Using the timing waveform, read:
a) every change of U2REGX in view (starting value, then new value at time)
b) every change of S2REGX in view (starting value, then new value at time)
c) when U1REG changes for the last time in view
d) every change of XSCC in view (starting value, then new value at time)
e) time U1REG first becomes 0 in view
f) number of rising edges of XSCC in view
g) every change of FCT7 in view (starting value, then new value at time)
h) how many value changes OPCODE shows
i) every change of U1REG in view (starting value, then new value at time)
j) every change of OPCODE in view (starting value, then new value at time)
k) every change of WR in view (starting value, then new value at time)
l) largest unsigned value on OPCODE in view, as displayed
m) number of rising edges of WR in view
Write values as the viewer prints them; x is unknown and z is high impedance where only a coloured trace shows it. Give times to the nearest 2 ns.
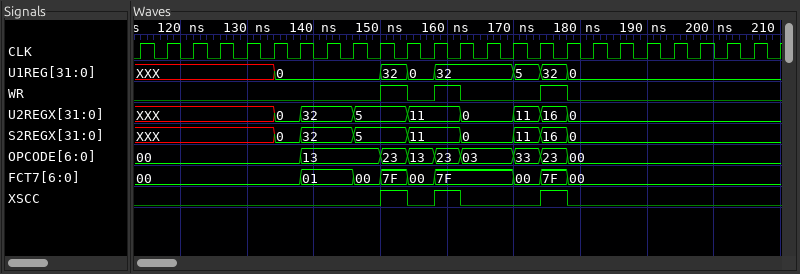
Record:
XXX, 0 at 134 ns, 32 at 138 ns, 5 at 146 ns, 11 at 154 ns, 0 at 162 ns, 11 at 170 ns, 16 at 174 ns, 0 at 178 ns
XXX, 0 at 134 ns, 32 at 138 ns, 5 at 146 ns, 11 at 154 ns, 0 at 162 ns, 11 at 170 ns, 16 at 174 ns, 0 at 178 ns
178 ns
0, 1 at 150 ns, 0 at 154 ns, 1 at 158 ns, 0 at 162 ns, 1 at 174 ns, 0 at 178 ns
134 ns
3
00, 01 at 138 ns, 00 at 146 ns, 7F at 150 ns, 00 at 154 ns, 7F at 158 ns, 00 at 170 ns, 7F at 174 ns, 00 at 178 ns
8
XXX, 0 at 134 ns, 32 at 150 ns, 0 at 154 ns, 32 at 158 ns, 5 at 170 ns, 32 at 174 ns, 0 at 178 ns
00, 13 at 138 ns, 23 at 150 ns, 13 at 154 ns, 23 at 158 ns, 03 at 162 ns, 33 at 170 ns, 23 at 174 ns, 00 at 178 ns
0, 1 at 150 ns, 0 at 154 ns, 1 at 158 ns, 0 at 162 ns, 1 at 174 ns, 0 at 178 ns
33
3
